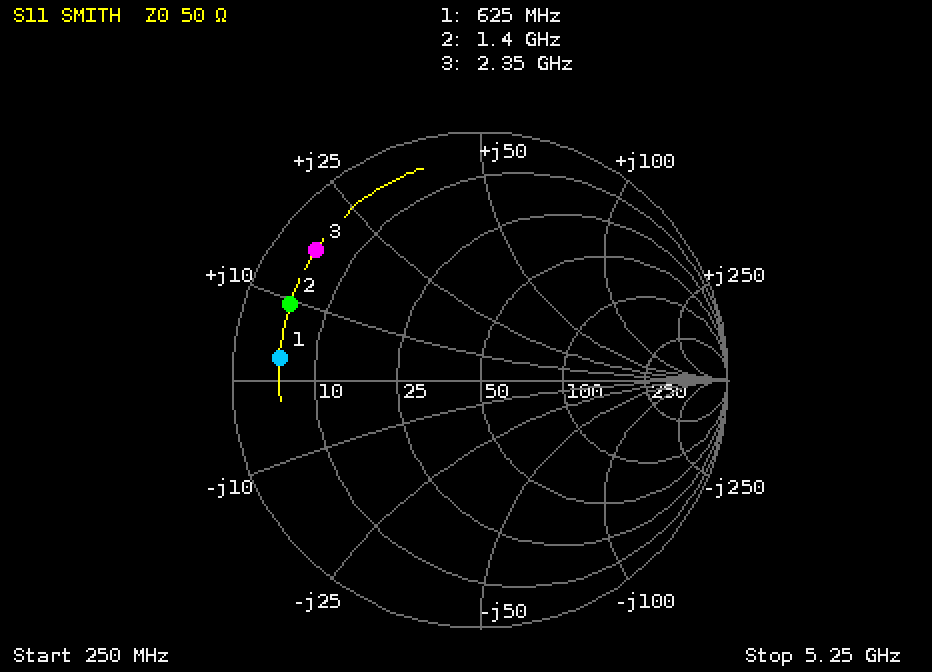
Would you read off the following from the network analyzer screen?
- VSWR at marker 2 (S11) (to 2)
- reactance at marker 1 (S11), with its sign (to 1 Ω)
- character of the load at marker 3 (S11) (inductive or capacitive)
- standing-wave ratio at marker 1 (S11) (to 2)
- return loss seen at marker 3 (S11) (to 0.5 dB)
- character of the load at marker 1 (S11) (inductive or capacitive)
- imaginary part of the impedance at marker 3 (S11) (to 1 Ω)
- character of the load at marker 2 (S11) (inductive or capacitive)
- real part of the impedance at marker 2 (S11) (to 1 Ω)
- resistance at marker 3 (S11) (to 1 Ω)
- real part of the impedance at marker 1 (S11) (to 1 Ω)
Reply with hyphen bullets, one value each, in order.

- 10
- +3 Ω
- inductive
- 10
- 1.5 dB
- inductive
- +17 Ω
- inductive
- 5 Ω
- 5 Ω
- 5 Ω
